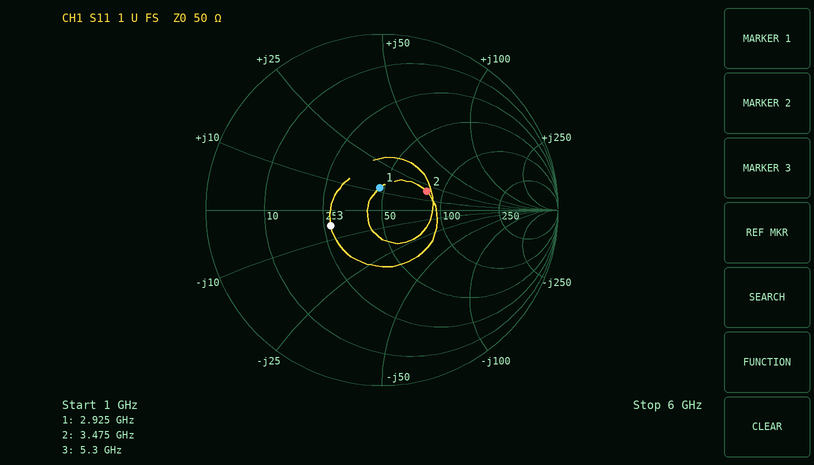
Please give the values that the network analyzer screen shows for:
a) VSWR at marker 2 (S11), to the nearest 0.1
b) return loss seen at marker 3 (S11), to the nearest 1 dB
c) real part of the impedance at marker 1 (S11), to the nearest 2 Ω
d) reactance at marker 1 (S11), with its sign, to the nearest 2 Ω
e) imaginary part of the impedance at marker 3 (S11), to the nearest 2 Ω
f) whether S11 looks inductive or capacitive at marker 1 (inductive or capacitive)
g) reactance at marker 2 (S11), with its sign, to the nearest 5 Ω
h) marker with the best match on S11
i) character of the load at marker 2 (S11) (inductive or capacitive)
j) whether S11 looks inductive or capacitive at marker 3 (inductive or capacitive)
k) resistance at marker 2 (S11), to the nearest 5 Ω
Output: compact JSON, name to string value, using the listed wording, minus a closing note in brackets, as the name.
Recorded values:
{"VSWR at marker 2 (S11), to the nearest 0.1": "1.8", "return loss seen at marker 3 (S11), to the nearest 1 dB": "10 dB", "real part of the impedance at marker 1 (S11), to the nearest 2 Ω": "48 Ω", "reactance at marker 1 (S11), with its sign, to the nearest 2 Ω": "+12 Ω", "imaginary part of the impedance at marker 3 (S11), to the nearest 2 Ω": "-6 Ω", "whether S11 looks inductive or capacitive at marker 1": "inductive", "reactance at marker 2 (S11), with its sign, to the nearest 5 Ω": "+20 Ω", "marker with the best match on S11": "marker 1", "character of the load at marker 2 (S11)": "inductive", "whether S11 looks inductive or capacitive at marker 3": "capacitive", "resistance at marker 2 (S11), to the nearest 5 Ω": "80 Ω"}
